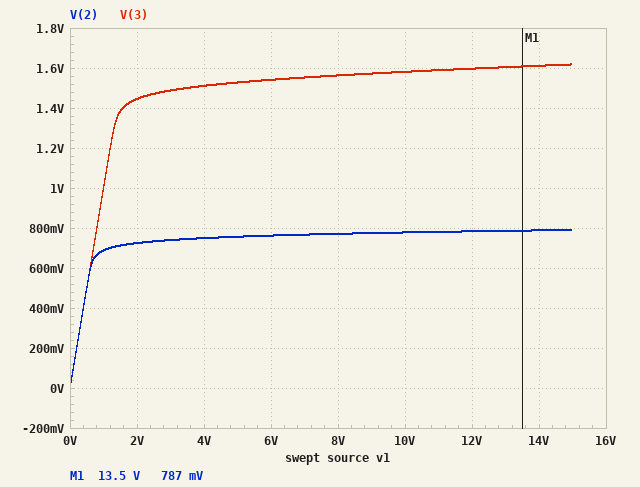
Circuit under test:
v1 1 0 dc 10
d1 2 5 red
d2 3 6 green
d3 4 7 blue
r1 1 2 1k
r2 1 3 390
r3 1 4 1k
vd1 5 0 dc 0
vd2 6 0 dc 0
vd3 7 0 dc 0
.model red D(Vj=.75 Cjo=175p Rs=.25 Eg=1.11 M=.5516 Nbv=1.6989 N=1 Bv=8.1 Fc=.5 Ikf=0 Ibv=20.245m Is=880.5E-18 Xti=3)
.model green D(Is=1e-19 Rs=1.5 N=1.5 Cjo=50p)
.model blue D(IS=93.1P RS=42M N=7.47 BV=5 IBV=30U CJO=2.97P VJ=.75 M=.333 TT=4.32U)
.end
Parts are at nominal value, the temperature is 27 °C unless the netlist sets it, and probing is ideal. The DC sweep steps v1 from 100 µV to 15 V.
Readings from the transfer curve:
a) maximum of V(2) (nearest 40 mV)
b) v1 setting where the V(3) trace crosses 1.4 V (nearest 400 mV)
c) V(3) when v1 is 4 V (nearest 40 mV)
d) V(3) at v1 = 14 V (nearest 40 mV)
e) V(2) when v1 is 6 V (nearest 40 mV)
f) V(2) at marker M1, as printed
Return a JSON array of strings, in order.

["800 mV", "1.6 V", "1.52 V", "1.60 V", "760 mV", "787 mV"]
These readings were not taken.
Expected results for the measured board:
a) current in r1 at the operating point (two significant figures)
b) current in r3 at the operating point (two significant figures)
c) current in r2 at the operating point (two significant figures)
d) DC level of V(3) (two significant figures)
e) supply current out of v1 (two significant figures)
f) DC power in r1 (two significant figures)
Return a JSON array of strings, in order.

["9.2 mA", "6.5 mA", "22 mA", "1.6 V", "37 mA", "85 mW"]
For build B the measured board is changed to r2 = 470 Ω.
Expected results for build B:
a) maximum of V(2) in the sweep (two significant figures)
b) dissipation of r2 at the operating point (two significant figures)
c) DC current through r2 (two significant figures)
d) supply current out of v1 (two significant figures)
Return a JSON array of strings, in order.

["790 mV", "150 mW", "18 mA", "34 mA"]
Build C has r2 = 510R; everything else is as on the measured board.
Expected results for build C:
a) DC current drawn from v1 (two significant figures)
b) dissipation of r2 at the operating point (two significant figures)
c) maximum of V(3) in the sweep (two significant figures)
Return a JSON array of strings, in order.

["32 mA", "140 mW", "1.6 V"]
